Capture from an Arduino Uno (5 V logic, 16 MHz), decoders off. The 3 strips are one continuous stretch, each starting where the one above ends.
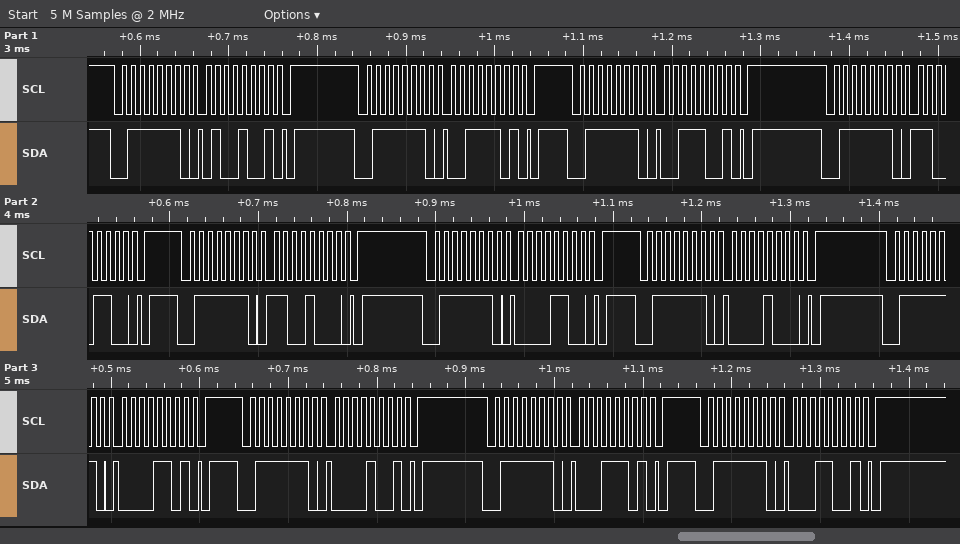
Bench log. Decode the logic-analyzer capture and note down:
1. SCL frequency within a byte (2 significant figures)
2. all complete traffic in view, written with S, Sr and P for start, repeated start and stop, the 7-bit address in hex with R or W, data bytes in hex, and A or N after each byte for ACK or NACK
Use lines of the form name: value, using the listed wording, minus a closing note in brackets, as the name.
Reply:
SCL frequency within a byte: 100 kHz
all complete traffic in view, written with S, Sr and P for start, repeated start and stop, the 7-bit address in hex with R or W, data bytes in hex, and A or N after each byte for ACK or NACK: S 3FW A 49 A P S 3FW A 3D A P S 3FW A 39 A P S 3FW A CC A P S 3FW A C8 A P S 3FW A 0C A P S 3FW A 08 A P S 3FW A 0D A P S 3FW A 09 A P S 3FW A 1D A P S 3FW A 19 A P
